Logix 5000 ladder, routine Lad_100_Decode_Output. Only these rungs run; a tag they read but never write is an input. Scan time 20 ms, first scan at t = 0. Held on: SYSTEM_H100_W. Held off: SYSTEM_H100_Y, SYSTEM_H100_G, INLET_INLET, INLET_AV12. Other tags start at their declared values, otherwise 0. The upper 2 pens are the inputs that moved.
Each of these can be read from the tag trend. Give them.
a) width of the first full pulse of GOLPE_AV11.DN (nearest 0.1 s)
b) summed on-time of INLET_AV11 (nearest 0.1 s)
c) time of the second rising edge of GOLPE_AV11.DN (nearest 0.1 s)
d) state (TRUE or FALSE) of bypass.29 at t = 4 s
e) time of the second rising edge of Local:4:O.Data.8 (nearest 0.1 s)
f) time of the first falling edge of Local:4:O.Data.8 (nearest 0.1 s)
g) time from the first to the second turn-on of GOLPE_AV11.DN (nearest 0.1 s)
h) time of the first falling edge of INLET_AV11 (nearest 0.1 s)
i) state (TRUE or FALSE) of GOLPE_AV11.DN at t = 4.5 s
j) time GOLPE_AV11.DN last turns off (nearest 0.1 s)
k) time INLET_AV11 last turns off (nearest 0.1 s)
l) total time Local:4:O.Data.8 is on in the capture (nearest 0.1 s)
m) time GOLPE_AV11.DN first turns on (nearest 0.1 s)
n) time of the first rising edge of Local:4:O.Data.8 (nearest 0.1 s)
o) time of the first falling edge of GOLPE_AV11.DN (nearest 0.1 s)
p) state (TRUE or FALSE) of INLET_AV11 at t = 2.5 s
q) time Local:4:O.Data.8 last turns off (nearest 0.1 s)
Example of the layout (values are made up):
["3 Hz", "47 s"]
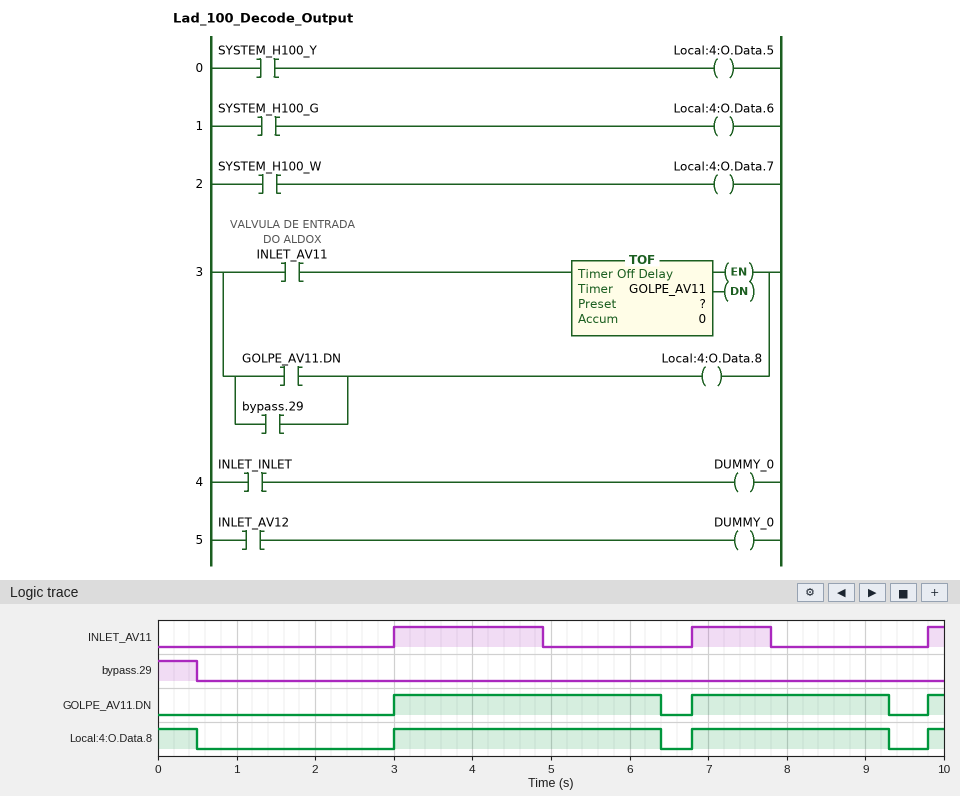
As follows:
["3.4 s", "3.1 s", "6.8 s", "FALSE", "6.8 s", "0.5 s", "3.8 s", "4.9 s", "TRUE", "9.3 s", "7.8 s", "6.6 s", "3.0 s", "3.0 s", "6.4 s", "FALSE", "9.3 s"]
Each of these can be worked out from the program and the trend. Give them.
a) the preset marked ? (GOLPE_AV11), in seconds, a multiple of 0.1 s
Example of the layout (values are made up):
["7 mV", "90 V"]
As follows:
["1.5 s"]
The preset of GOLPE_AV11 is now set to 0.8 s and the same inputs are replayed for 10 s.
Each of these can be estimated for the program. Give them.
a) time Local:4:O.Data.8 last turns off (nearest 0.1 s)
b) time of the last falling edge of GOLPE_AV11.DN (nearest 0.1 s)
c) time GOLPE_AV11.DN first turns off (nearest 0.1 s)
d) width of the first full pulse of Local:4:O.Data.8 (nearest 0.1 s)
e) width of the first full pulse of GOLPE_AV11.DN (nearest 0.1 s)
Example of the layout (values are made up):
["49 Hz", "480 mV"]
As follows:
["8.6 s", "8.6 s", "5.7 s", "2.7 s", "2.7 s"]
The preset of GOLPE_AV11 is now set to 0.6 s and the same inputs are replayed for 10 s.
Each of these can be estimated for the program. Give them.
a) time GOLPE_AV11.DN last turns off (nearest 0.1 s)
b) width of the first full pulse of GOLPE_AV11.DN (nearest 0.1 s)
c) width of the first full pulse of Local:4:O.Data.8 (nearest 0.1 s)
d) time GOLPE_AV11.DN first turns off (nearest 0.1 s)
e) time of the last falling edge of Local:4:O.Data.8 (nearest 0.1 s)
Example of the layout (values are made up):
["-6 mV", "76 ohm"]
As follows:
["8.4 s", "2.5 s", "2.5 s", "5.5 s", "8.4 s"]
